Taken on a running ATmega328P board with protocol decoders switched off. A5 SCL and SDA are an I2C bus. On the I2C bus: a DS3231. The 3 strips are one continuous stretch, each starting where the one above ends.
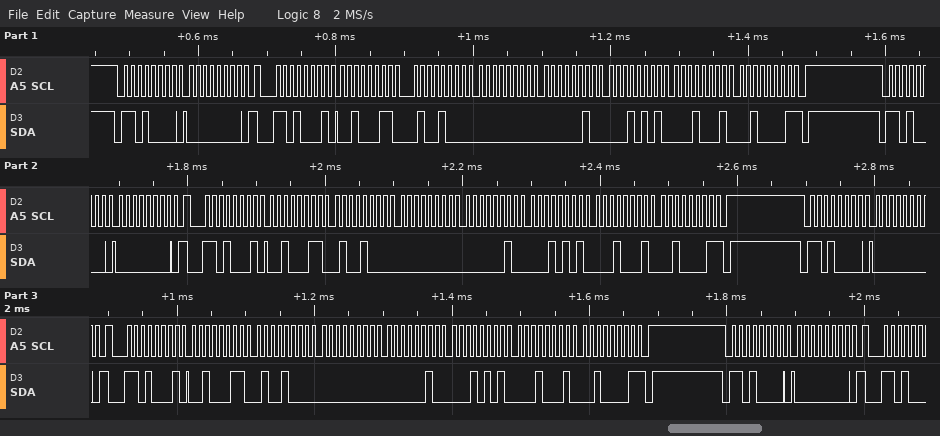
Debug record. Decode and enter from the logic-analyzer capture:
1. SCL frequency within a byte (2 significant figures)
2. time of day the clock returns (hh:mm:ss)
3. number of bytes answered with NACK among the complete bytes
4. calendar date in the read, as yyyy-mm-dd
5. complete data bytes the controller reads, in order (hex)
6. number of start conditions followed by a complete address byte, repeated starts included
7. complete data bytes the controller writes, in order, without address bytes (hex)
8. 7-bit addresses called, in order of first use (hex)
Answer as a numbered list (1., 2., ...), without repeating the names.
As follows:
1. 100 kHz
2. 00:48:23
3. 3
4. 2021-11-15
5. 23 48 00 02 15 11 21 23 48 00 02 15 11 21 23 48 00 02 15 11 21
6. 7
7. 00 00 00 00
8. 0x68
